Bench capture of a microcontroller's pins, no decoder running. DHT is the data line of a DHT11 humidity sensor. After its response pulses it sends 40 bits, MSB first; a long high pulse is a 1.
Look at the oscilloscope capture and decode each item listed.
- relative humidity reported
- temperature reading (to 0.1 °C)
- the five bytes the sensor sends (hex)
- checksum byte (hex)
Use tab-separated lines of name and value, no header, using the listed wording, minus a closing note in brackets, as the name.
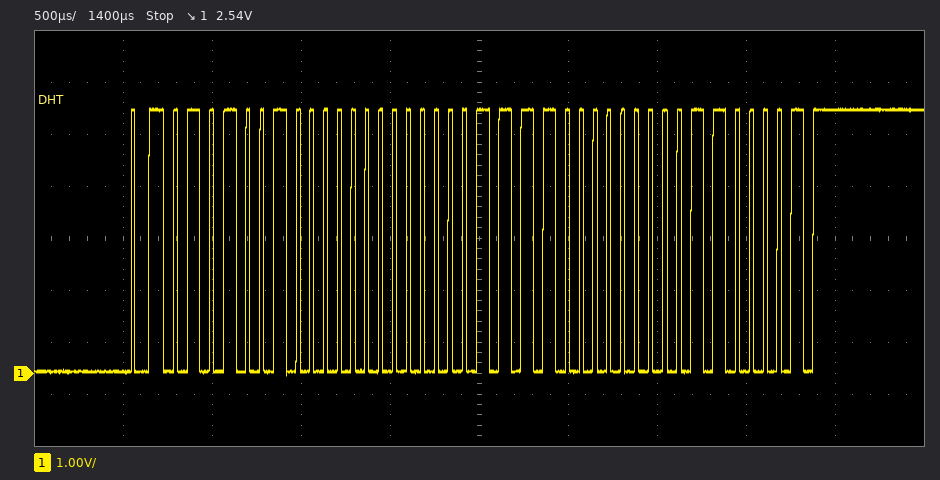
relative humidity reported	82 %
temperature reading	15.0 °C
the five bytes the sensor sends	52 00 0F 00 61
checksum byte	0x61
